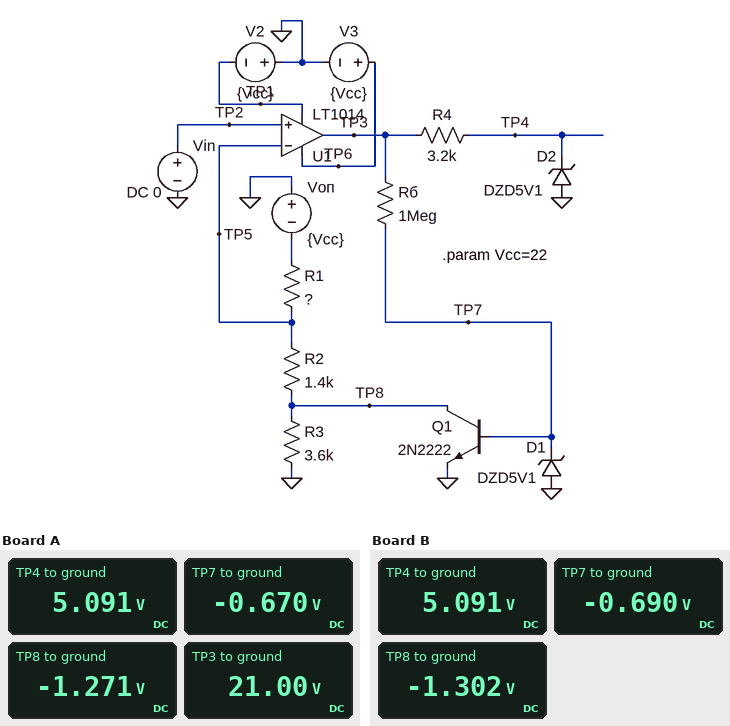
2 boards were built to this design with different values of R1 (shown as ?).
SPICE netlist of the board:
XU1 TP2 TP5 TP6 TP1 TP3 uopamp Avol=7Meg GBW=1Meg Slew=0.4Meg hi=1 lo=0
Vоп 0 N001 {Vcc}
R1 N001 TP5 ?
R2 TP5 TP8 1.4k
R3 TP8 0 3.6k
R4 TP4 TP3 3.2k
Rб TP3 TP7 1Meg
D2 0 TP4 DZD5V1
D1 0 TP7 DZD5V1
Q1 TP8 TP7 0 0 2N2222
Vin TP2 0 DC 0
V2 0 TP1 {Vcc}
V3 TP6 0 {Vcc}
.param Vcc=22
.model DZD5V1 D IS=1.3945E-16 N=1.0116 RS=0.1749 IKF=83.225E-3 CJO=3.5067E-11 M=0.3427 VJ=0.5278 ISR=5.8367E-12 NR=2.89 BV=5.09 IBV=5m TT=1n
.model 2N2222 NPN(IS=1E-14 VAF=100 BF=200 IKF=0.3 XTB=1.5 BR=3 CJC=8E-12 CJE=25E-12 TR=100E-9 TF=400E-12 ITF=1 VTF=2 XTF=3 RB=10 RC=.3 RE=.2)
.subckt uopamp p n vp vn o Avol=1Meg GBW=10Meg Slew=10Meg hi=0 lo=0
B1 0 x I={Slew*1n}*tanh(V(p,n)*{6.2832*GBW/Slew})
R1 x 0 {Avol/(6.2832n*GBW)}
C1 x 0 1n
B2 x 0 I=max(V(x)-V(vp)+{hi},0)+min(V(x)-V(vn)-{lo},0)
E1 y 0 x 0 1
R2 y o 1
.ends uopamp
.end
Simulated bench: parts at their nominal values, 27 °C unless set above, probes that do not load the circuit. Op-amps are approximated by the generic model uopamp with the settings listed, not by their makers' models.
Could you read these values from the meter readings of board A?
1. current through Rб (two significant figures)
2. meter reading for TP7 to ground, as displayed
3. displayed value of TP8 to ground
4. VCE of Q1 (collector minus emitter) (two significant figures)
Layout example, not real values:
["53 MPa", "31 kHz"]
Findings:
["22 µA", "-0.670 V", "-1.271 V", "-1.3 V"]
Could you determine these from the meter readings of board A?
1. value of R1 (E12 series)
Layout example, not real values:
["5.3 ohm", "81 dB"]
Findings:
["39 kΩ"]
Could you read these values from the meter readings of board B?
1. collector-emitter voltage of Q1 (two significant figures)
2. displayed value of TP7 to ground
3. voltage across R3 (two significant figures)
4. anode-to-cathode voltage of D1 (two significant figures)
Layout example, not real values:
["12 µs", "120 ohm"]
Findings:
["-1.3 V", "-0.690 V", "1.3 V", "690 mV"]
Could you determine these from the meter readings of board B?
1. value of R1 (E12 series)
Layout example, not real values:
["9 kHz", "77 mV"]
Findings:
["33 kΩ"]
